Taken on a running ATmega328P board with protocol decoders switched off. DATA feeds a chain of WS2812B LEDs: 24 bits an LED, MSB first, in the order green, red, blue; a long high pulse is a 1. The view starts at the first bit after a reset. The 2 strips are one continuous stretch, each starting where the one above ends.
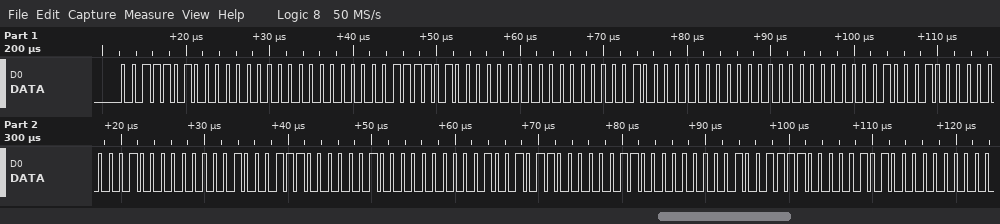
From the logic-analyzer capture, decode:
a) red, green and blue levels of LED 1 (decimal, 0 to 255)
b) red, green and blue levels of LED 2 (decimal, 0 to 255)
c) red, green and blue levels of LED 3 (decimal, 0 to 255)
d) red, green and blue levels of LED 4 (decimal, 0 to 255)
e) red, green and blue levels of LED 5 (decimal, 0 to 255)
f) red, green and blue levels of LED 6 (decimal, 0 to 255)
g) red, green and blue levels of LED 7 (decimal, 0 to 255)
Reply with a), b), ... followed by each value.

a) 0, 58, 0
b) 0, 61, 0
c) 0, 64, 0
d) 1, 68, 0
e) 2, 71, 0
f) 3, 75, 0
g) 5, 79, 0
